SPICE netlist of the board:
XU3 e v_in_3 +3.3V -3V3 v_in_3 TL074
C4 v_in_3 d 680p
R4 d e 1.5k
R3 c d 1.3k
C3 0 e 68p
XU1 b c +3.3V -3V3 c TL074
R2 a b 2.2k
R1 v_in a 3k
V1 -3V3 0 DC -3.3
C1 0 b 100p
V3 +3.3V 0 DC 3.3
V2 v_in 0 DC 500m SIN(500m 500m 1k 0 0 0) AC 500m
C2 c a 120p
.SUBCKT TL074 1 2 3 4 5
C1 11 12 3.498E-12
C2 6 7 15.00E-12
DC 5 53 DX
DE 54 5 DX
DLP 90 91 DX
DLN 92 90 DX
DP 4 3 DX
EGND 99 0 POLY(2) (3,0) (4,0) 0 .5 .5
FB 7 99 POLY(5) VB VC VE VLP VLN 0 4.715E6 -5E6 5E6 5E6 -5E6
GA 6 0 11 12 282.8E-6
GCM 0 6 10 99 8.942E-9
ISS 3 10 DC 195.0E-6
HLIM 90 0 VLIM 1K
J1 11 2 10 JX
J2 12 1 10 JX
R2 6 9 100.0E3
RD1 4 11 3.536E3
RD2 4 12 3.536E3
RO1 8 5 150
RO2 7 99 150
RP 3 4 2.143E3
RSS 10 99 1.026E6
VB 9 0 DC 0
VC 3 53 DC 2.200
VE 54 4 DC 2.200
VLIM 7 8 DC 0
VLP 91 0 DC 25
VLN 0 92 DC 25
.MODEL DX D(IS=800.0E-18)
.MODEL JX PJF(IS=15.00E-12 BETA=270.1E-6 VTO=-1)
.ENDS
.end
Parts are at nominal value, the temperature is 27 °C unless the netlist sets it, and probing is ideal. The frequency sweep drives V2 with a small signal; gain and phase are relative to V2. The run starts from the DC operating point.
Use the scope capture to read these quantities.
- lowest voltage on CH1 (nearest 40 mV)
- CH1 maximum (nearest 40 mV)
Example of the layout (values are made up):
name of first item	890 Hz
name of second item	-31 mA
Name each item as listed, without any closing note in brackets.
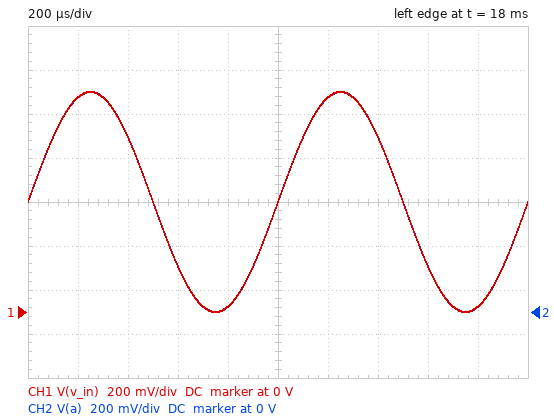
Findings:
lowest voltage on CH1	0 V
CH1 maximum	1.00 V
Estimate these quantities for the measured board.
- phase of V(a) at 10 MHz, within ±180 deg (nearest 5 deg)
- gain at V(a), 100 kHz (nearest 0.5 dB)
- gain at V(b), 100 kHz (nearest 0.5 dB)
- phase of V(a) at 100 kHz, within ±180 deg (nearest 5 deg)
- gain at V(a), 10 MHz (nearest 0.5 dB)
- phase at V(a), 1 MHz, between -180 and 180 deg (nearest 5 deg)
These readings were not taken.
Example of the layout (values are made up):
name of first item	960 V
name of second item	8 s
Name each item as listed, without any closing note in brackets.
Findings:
phase of V(a) at 10 MHz, within ±180 deg	-30 deg
gain at V(a), 100 kHz	0 dB
gain at V(b), 100 kHz	0 dB
phase of V(a) at 100 kHz, within ±180 deg	-10 deg
gain at V(a), 10 MHz	-25.0 dB
phase at V(a), 1 MHz, between -180 and 180 deg	-75 deg
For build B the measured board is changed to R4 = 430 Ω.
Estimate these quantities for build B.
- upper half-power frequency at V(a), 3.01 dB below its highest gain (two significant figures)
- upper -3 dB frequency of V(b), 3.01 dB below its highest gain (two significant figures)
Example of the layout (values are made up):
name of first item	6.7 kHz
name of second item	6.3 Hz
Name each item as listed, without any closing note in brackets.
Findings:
upper half-power frequency at V(a), 3.01 dB below its highest gain	550 kHz
upper -3 dB frequency of V(b), 3.01 dB below its highest gain	420 kHz
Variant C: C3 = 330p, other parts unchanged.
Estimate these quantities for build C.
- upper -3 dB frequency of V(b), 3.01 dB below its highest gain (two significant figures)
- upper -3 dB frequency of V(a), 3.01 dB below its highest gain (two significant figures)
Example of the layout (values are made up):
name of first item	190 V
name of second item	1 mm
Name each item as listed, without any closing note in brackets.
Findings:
upper -3 dB frequency of V(b), 3.01 dB below its highest gain	420 kHz
upper -3 dB frequency of V(a), 3.01 dB below its highest gain	530 kHz
